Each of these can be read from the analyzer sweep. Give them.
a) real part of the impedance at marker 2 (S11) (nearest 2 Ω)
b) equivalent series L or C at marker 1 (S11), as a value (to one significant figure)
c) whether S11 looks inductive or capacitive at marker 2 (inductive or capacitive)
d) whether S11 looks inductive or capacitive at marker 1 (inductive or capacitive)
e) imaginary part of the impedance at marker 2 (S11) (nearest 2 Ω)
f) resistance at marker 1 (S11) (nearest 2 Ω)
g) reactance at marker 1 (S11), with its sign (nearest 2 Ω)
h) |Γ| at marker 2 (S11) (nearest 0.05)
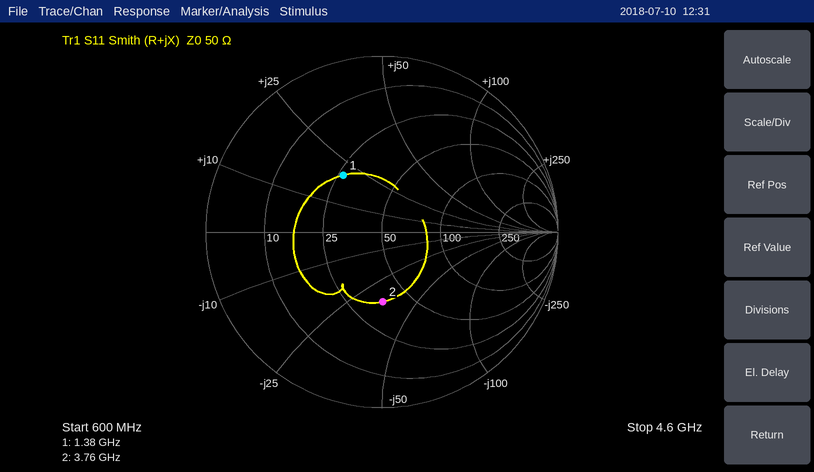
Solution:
36 Ω
2 nH
capacitive
inductive
-34 Ω
26 Ω
+20 Ω
0.40
